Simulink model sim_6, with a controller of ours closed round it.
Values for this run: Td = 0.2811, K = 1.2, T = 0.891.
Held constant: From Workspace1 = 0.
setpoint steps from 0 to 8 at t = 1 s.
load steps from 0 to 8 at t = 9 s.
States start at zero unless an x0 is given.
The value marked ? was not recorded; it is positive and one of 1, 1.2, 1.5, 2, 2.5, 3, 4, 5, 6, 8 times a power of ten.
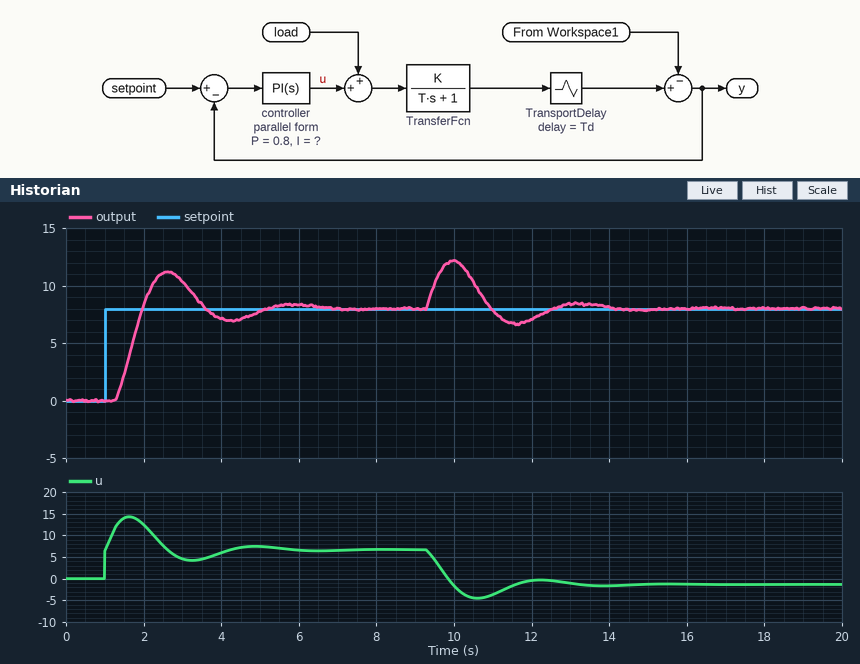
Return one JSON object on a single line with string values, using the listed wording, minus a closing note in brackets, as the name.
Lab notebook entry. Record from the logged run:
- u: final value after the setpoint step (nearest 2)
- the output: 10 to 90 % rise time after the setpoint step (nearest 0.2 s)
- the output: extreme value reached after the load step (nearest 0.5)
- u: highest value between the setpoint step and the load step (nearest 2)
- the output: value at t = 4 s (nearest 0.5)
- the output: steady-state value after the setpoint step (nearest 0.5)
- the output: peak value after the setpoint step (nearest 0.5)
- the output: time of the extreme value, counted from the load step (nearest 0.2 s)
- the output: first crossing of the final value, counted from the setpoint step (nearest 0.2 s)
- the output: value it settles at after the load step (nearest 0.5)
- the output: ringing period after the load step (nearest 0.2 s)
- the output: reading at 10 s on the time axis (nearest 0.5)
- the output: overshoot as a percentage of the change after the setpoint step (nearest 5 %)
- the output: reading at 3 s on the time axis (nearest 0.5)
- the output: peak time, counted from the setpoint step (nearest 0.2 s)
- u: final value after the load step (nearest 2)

{"u: final value after the setpoint step": "6", "the output: 10 to 90 % rise time after the setpoint step": "0.6 s", "the output: extreme value reached after the load step": "12.0", "u: highest value between the setpoint step and the load step": "14", "the output: value at t = 4 s": "7.0", "the output: steady-state value after the setpoint step": "8.0", "the output: peak value after the setpoint step": "11.0", "the output: time of the extreme value, counted from the load step": "1.0 s", "the output: first crossing of the final value, counted from the setpoint step": "1.0 s", "the output: value it settles at after the load step": "8.0", "the output: ringing period after the load step": "3.2 s", "the output: reading at 10 s on the time axis": "12.0", "the output: overshoot as a percentage of the change after the setpoint step": "40 %", "the output: reading at 3 s on the time axis": "10.5", "the output: peak time, counted from the setpoint step": "1.6 s", "u: final value after the load step": "-2"}
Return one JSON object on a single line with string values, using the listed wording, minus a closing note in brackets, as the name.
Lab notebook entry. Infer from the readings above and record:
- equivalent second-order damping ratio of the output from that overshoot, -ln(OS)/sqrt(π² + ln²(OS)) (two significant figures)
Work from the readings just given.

{"equivalent second-order damping ratio of the output from that overshoot, -ln(OS)/sqrt(π² + ln²(OS))": "0.28"}
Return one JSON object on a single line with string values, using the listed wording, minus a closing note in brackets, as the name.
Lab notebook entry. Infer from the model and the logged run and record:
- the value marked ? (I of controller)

{"the value marked ?": "2.5"}
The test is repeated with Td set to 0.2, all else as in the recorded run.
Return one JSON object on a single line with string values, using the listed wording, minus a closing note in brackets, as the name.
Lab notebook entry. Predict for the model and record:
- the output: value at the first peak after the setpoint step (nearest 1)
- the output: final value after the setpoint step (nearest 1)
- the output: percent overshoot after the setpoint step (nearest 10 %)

{"the output: value at the first peak after the setpoint step": "10", "the output: final value after the setpoint step": "8", "the output: percent overshoot after the setpoint step": "30 %"}
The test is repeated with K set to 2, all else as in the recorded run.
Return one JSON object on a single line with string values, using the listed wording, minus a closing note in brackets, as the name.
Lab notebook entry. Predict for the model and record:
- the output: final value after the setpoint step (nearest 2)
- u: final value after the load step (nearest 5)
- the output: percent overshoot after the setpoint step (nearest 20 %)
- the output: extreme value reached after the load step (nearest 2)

{"the output: final value after the setpoint step": "8", "u: final value after the load step": "-5", "the output: percent overshoot after the setpoint step": "60 %", "the output: extreme value reached after the load step": "14"}
